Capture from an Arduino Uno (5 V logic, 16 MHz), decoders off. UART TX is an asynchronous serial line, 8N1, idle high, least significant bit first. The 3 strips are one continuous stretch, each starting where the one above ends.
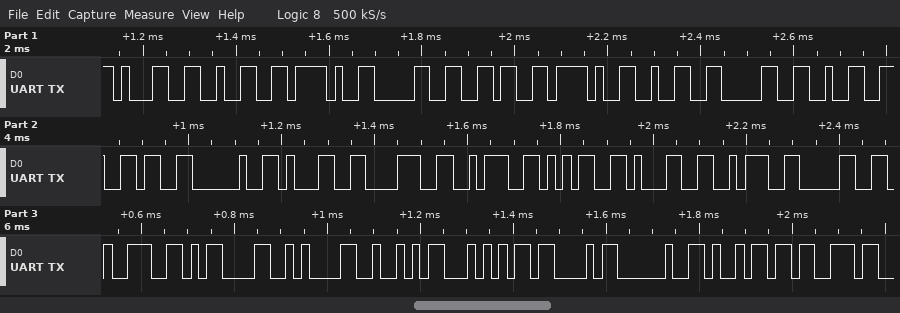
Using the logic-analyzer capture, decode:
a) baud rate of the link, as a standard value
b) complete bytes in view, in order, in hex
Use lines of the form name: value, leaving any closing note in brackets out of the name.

baud rate of the link, as a standard value: 57600 baud
complete bytes in view, in order, in hex: 31 32 2F 30 36 2F 32 30 32 36 20 31 38 3A 35 31 3A 30 39 0D 0A 52 54 43 20 69 73
